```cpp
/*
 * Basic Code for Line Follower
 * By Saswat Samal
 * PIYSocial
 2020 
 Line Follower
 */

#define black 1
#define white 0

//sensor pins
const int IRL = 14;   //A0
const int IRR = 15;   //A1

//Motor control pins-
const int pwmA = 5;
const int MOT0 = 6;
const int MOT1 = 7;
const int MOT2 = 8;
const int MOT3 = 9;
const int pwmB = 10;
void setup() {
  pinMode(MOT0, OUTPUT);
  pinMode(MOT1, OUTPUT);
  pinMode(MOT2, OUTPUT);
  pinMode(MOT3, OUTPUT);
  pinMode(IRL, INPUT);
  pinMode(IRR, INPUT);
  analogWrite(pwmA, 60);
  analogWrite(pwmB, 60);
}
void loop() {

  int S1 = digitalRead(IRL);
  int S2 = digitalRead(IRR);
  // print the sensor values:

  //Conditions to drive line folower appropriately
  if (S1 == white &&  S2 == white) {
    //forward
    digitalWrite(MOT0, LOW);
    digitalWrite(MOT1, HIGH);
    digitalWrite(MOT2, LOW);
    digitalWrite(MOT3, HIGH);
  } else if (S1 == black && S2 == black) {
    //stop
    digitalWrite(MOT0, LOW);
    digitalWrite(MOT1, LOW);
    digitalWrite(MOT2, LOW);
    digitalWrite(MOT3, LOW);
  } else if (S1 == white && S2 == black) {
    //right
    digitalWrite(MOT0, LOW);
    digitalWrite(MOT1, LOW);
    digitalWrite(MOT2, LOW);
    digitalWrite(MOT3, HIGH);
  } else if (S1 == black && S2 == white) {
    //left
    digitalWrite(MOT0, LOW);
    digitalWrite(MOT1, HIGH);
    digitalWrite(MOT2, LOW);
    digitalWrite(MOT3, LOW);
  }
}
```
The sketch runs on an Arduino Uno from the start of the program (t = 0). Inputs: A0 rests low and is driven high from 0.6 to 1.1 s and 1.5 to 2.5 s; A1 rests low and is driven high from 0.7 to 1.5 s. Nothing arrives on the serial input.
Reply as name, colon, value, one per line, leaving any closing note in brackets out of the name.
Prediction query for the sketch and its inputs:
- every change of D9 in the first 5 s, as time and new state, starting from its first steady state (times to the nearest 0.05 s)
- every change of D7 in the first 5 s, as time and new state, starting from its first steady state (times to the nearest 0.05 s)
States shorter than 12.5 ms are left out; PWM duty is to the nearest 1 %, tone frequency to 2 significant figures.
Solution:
every change of D9 in the first 5 s, as time and new state, starting from its first steady state: 0 s high; 0.6 s low; 1.1 s high; 1.5 s low; 2.5 s high
every change of D7 in the first 5 s, as time and new state, starting from its first steady state: 0 s high; 0.7 s low; 1.5 s high
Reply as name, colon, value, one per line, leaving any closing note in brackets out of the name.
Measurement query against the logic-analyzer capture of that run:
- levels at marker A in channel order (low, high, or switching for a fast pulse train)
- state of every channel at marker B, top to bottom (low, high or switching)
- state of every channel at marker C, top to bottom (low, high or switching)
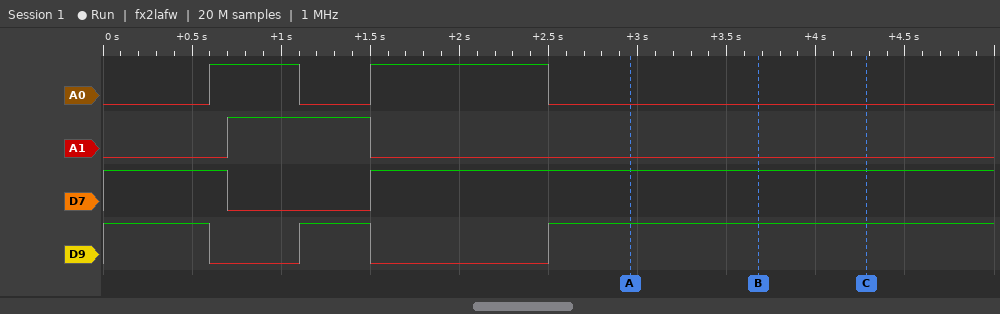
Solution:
levels at marker A in channel order: A0 low, A1 low, D7 high, D9 high
state of every channel at marker B, top to bottom: A0 low, A1 low, D7 high, D9 high
state of every channel at marker C, top to bottom: A0 low, A1 low, D7 high, D9 high
